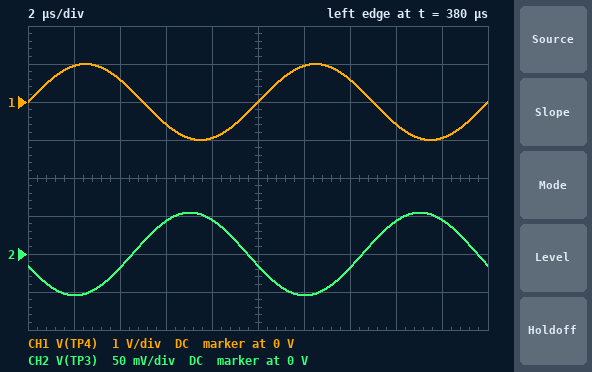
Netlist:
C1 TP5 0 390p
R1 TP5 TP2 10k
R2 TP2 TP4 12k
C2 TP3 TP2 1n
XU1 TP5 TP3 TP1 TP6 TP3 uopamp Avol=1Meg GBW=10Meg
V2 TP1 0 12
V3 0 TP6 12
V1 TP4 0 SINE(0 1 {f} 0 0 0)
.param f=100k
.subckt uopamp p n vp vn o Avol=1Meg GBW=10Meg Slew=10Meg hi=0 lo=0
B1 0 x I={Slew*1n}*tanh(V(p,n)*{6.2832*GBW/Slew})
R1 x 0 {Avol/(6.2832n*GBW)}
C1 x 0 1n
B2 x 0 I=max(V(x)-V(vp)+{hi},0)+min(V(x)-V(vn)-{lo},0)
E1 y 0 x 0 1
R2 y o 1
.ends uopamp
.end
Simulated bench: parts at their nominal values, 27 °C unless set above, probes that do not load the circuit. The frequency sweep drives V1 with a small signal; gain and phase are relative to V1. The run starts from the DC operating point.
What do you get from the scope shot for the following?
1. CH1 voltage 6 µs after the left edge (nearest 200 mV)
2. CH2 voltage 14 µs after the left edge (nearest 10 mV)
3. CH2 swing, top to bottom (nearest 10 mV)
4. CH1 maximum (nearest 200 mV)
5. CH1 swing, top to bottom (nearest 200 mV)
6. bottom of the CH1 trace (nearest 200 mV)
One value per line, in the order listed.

-600 mV
-20 mV
110 mV
1.0 V
2.0 V
-1.0 V
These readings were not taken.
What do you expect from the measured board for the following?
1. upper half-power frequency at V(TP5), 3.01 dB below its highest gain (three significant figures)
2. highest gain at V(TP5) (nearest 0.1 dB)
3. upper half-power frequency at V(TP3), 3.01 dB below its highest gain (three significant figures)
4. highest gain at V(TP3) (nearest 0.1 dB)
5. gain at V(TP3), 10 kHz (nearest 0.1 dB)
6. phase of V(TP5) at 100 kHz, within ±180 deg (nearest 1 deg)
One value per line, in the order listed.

25.4 kHz
0.2 dB
25.4 kHz
0.2 dB
0.2 dB
-163 deg
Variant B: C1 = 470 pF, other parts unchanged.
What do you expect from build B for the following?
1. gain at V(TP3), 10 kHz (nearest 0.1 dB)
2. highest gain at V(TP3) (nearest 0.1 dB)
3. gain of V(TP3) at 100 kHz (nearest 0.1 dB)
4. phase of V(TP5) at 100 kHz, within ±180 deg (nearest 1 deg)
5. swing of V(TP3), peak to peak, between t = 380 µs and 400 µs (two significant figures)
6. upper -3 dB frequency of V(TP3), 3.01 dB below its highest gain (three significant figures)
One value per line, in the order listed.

-0.1 dB
0 dB
-27.0 dB
-163 deg
90 mV
21.7 kHz
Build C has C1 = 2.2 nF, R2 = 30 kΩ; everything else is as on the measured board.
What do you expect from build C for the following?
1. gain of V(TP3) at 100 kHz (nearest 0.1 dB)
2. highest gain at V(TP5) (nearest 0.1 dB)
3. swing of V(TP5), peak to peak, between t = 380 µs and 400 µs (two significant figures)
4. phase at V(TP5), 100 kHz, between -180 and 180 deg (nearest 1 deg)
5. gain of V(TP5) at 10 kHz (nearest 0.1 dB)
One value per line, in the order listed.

-48.5 dB
0 dB
7.5 mV
-168 deg
-15.2 dB
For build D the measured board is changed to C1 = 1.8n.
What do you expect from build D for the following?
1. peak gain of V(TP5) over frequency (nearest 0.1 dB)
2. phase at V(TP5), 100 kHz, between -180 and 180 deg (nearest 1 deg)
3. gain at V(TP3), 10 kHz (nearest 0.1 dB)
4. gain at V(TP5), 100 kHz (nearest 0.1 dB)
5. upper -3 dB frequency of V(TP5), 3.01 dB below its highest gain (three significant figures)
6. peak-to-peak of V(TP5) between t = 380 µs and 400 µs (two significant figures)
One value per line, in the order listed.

0 dB
-164 deg
-7.9 dB
-38.9 dB
4.64 kHz
23 mV
